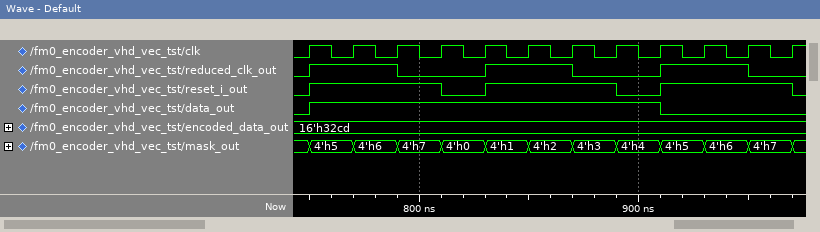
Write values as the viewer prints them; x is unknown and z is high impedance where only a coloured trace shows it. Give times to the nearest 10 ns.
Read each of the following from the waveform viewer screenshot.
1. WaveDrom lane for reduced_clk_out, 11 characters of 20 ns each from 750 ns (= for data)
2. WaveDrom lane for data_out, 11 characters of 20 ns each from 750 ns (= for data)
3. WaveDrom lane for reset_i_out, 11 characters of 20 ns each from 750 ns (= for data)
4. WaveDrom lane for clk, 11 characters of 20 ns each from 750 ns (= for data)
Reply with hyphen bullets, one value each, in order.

- {name: 'reduced_clk_out', wave: '1.0.1.0.1.0'}
- {name: 'data_out', wave: '1.......0..'}
- {name: 'reset_i_out', wave: '1..01..01..'}
- {name: 'clk', wave: 'p..........'}
